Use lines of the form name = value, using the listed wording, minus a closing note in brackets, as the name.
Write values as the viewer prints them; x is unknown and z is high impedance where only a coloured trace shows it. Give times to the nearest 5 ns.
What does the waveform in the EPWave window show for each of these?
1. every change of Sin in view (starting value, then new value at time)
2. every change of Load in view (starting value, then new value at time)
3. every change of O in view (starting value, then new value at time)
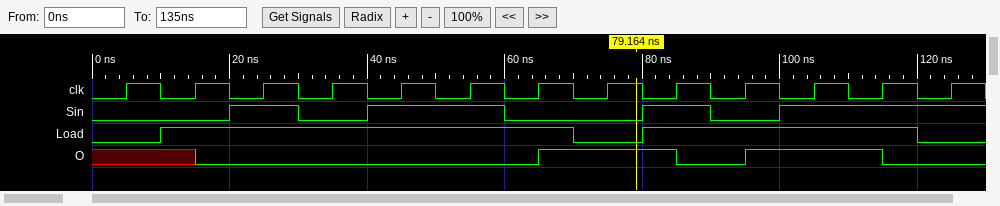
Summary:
every change of Sin in view = 0, 1 at 20 ns, 0 at 30 ns, 1 at 40 ns, 0 at 60 ns, 1 at 80 ns, 0 at 90 ns, 1 at 100 ns
every change of Load in view = 0, 1 at 10 ns, 0 at 70 ns, 1 at 80 ns, 0 at 120 ns
every change of O in view = x, 0 at 15 ns, 1 at 65 ns, 0 at 85 ns, 1 at 95 ns, 0 at 115 ns
